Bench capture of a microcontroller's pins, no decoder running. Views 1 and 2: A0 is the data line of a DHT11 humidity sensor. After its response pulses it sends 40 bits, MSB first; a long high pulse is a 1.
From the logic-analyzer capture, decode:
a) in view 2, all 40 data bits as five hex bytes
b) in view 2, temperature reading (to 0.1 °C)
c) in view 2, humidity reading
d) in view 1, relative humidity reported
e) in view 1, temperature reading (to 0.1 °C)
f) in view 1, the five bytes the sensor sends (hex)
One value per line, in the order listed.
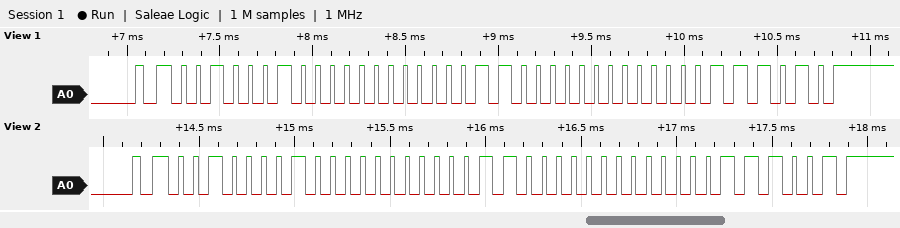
21 00 18 00 39
24.0 °C
33 %
34 %
24.0 °C
22 00 18 00 3A
